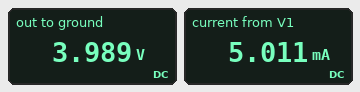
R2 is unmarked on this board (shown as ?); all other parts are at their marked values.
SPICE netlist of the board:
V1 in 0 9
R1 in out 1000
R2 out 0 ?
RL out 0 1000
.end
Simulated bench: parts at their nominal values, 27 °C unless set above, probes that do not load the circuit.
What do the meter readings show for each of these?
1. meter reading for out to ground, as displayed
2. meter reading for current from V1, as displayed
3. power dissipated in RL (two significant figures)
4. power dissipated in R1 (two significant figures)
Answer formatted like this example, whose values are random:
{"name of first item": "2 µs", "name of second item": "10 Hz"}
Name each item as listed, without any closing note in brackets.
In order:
{"meter reading for out to ground, as displayed": "3.989 V", "meter reading for current from V1, as displayed": "5.011 mA", "power dissipated in RL": "16 mW", "power dissipated in R1": "25 mW"}
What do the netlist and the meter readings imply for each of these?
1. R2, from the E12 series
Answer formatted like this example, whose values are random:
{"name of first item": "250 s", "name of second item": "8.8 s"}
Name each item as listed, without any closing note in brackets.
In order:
{"R2, from the E12 series": "3.9 kΩ"}
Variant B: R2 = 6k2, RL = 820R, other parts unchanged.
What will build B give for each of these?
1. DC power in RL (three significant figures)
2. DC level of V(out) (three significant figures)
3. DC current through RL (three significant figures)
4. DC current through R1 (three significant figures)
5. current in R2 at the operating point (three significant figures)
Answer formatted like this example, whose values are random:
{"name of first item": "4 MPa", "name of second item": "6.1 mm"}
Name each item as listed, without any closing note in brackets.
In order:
{"DC power in RL": "17.4 mW", "DC level of V(out)": "3.78 V", "DC current through RL": "4.61 mA", "DC current through R1": "5.22 mA", "current in R2 at the operating point": "610 µA"}
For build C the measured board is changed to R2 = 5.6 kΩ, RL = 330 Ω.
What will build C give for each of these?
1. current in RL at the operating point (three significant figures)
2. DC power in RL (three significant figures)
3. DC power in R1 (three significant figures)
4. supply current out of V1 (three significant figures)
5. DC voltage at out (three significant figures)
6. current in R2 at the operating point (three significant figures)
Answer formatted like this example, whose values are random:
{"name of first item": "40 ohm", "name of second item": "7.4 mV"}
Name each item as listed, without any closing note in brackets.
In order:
{"current in RL at the operating point": "6.48 mA", "DC power in RL": "13.9 mW", "DC power in R1": "47.1 mW", "supply current out of V1": "6.86 mA", "DC voltage at out": "2.14 V", "current in R2 at the operating point": "382 µA"}
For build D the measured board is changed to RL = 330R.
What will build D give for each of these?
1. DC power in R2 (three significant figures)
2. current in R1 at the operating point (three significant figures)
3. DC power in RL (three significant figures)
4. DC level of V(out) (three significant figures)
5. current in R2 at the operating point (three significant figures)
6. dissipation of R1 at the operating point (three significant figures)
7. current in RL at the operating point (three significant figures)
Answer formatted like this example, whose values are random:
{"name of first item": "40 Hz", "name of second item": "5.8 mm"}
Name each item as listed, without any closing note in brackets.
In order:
{"DC power in R2": "1.13 mW", "current in R1 at the operating point": "6.90 mA", "DC power in RL": "13.4 mW", "DC level of V(out)": "2.10 V", "current in R2 at the operating point": "538 µA", "dissipation of R1 at the operating point": "47.6 mW", "current in RL at the operating point": "6.36 mA"}
